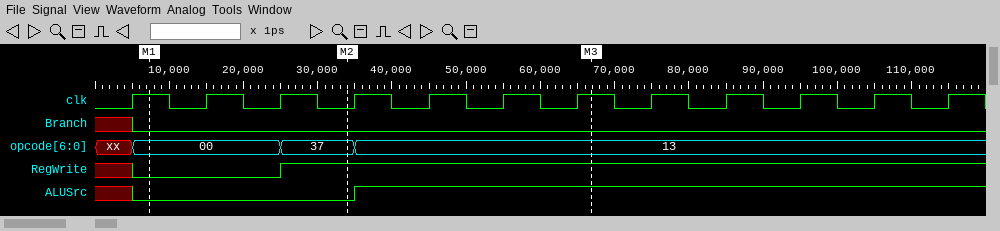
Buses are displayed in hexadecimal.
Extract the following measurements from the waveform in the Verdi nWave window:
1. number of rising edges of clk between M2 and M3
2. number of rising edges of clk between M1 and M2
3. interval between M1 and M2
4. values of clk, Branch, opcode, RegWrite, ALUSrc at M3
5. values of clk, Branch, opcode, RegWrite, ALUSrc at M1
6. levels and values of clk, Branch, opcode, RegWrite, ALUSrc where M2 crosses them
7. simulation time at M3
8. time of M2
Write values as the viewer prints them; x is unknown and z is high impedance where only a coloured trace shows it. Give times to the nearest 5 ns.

4
2
25 ns
clk=1, Branch=0, opcode=13, RegWrite=1, ALUSrc=1
clk=1, Branch=0, opcode=00, RegWrite=0, ALUSrc=0
clk=0, Branch=0, opcode=37, RegWrite=1, ALUSrc=0
65 ns
35 ns
